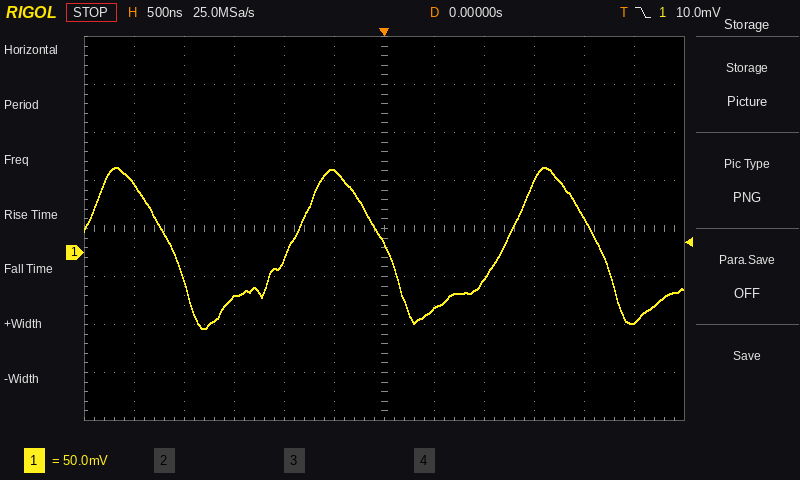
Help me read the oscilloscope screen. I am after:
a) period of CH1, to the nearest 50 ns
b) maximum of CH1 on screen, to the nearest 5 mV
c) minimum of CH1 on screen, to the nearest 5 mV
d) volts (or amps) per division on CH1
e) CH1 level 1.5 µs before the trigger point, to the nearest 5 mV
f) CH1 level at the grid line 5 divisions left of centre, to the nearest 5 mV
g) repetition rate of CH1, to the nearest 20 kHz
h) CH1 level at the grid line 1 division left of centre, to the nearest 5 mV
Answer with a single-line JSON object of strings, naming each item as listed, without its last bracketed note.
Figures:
{"period of CH1, to the nearest 50 ns": "2.15 µs", "maximum of CH1 on screen, to the nearest 5 mV": "90 mV", "minimum of CH1 on screen, to the nearest 5 mV": "-80 mV", "volts (or amps) per division on CH1": "50 mV", "CH1 level 1.5 µs before the trigger point, to the nearest 5 mV": "-45 mV", "CH1 level at the grid line 5 divisions left of centre, to the nearest 5 mV": "70 mV", "repetition rate of CH1, to the nearest 20 kHz": "460 kHz", "CH1 level at the grid line 1 division left of centre, to the nearest 5 mV": "85 mV"}
